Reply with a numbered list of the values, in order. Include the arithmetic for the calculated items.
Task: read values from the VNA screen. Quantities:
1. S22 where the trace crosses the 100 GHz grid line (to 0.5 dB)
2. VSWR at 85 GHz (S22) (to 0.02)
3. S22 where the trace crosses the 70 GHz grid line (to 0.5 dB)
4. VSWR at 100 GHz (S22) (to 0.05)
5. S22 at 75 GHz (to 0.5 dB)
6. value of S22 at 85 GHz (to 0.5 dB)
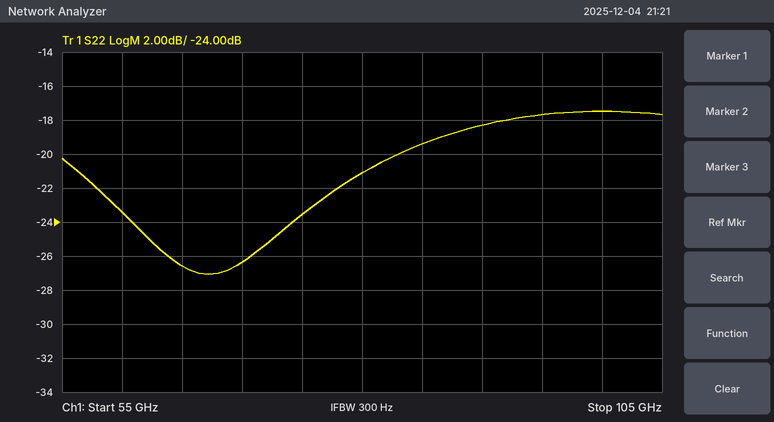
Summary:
1. -17.5 dB
2. |Γ| = 10^(-19.5/20) = 0.1059; VSWR = (1 + 0.1059)/(1 − 0.1059) ≈ 1.24
3. -26.5 dB
4. |Γ| = 10^(-17.5/20) = 0.1334; VSWR = (1 + 0.1334)/(1 − 0.1334) ≈ 1.31, so 1.30 to the nearest 0.05
5. -23.5 dB
6. -19.5 dB
